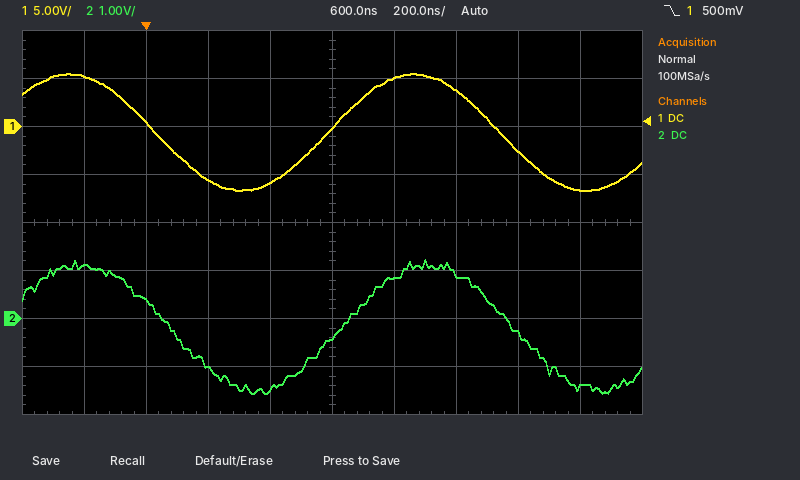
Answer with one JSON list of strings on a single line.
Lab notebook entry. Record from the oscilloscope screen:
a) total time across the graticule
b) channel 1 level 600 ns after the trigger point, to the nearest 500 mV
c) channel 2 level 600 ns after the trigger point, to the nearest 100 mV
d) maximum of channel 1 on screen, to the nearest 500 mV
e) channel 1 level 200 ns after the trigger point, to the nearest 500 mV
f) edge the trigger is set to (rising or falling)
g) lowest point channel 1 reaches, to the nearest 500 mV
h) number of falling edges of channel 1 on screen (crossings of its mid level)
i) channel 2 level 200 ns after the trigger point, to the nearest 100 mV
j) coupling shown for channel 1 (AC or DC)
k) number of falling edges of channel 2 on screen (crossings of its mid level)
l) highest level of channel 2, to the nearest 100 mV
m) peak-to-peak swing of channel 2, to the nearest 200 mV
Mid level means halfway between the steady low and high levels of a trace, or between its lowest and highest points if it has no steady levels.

["2 µs", "0.0 V", "-400 mV", "5.5 V", "-5.5 V", "falling", "-6.5 V", "2", "-1.0 V", "DC", "2", "1.2 V", "2.8 V"]
